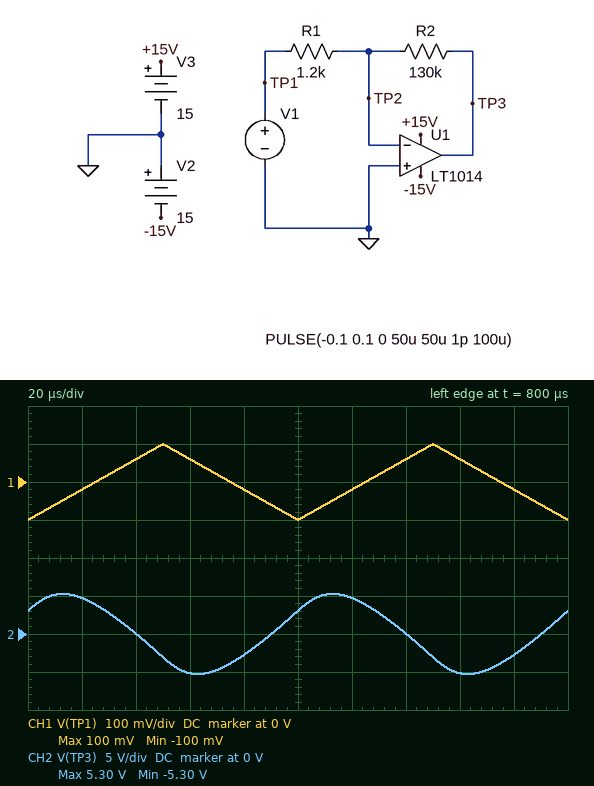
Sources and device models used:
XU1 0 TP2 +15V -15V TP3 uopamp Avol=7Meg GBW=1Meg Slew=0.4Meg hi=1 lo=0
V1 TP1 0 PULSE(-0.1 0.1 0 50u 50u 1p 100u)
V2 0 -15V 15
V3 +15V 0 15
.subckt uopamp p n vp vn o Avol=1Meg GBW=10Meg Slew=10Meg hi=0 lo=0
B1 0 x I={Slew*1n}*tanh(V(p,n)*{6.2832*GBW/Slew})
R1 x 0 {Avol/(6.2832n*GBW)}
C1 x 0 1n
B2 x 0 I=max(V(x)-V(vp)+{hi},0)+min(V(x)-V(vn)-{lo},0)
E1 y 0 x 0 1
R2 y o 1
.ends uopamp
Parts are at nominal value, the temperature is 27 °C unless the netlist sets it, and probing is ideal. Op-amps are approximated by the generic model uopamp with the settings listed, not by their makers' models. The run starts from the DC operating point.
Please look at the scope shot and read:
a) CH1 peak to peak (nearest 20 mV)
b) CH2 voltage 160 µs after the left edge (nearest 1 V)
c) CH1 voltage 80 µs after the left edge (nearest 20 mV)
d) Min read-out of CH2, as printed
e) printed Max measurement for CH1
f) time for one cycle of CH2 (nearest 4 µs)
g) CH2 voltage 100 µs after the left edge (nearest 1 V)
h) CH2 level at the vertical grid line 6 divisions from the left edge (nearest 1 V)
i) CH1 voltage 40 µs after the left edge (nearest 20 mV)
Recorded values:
200 mV
-5 V
-20 mV
-5.30 V
100 mV
100 µs
3 V
5 V
60 mV
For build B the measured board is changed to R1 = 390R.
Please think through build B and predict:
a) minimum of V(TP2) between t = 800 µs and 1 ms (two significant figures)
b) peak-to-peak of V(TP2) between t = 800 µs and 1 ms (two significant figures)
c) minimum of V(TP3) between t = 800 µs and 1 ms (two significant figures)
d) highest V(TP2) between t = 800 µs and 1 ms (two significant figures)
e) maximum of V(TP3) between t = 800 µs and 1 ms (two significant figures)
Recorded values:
-96 mV
190 mV
-5.8 V
96 mV
5.8 V
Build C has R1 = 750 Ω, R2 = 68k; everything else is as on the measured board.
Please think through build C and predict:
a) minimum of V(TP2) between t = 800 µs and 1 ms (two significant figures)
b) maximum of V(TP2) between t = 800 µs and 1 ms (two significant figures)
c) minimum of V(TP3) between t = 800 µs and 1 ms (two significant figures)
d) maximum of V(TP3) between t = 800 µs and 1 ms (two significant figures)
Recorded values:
-63 mV
63 mV
-5.0 V
5.0 V
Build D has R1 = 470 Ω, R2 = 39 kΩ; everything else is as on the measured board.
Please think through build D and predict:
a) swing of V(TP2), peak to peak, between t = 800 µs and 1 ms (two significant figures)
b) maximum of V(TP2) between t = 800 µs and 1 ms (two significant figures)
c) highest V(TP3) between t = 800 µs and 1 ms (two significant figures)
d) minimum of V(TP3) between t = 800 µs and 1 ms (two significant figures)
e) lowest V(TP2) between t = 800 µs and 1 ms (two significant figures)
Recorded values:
120 mV
58 mV
4.9 V
-4.9 V
-58 mV
